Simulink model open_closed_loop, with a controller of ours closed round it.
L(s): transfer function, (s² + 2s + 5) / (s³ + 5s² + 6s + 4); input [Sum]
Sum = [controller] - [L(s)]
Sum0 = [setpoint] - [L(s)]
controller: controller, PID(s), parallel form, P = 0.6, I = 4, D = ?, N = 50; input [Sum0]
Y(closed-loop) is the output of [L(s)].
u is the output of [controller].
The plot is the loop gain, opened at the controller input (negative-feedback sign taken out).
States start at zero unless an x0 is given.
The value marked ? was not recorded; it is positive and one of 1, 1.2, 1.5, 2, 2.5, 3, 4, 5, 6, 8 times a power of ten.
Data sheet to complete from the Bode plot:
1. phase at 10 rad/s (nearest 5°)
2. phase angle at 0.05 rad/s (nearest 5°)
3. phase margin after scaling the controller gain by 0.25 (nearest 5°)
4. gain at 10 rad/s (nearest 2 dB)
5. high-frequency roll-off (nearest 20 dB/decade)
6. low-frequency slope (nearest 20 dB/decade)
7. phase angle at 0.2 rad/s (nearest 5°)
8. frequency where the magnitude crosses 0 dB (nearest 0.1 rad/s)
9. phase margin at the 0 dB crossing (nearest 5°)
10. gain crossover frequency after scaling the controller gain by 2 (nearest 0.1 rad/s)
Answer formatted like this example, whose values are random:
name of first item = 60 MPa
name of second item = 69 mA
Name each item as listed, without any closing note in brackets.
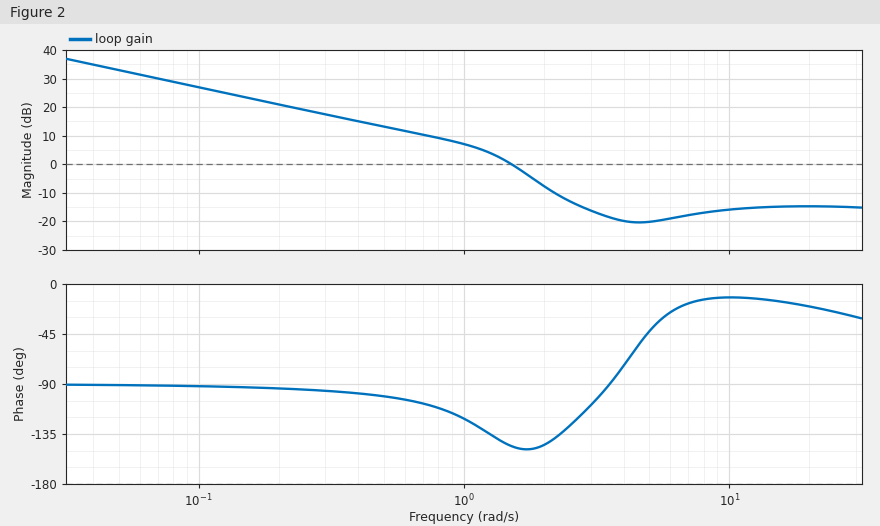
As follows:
phase at 10 rad/s = -10°
phase angle at 0.05 rad/s = -90°
phase margin after scaling the controller gain by 0.25 = 75°
gain at 10 rad/s = -16 dB
high-frequency roll-off = 0 dB/decade
low-frequency slope = -20 dB/decade
phase angle at 0.2 rad/s = -95°
frequency where the magnitude crosses 0 dB = 1.5 rad/s
phase margin at the 0 dB crossing = 35°
gain crossover frequency after scaling the controller gain by 2 = 1.9 rad/s
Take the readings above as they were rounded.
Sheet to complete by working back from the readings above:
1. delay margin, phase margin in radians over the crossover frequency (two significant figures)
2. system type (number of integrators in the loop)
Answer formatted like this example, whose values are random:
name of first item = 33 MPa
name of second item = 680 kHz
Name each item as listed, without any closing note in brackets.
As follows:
delay margin, phase margin in radians over the crossover frequency = 0.41 s
system type = 1
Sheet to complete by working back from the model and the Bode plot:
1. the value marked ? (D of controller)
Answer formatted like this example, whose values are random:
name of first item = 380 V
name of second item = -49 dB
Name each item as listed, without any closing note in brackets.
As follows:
the value marked ? = 0.2
